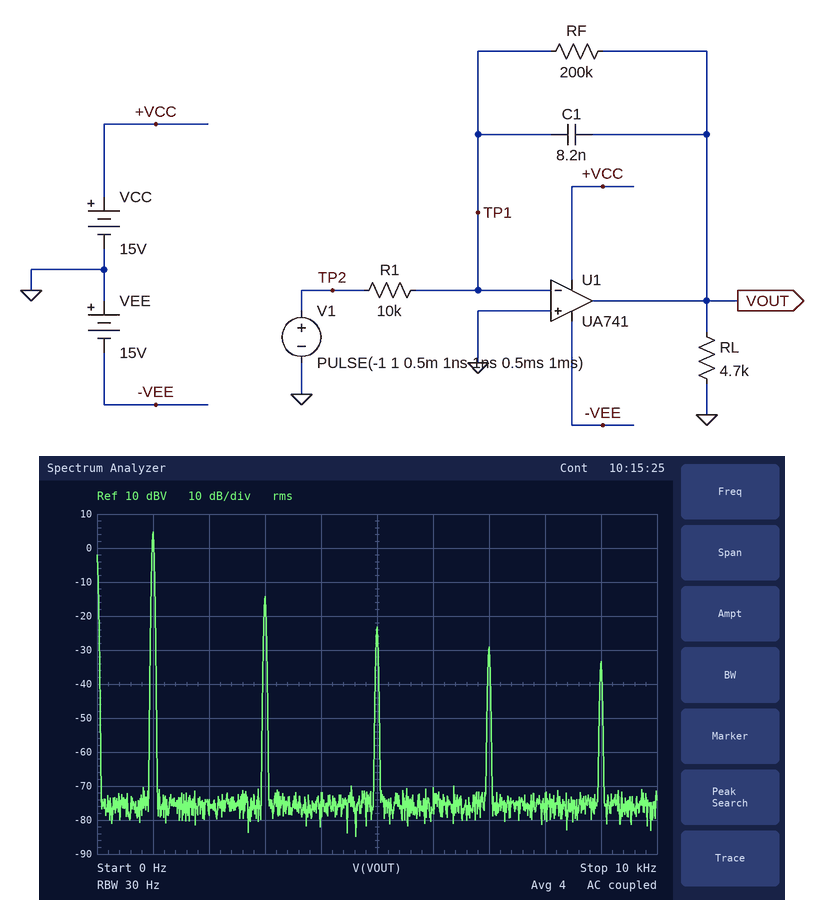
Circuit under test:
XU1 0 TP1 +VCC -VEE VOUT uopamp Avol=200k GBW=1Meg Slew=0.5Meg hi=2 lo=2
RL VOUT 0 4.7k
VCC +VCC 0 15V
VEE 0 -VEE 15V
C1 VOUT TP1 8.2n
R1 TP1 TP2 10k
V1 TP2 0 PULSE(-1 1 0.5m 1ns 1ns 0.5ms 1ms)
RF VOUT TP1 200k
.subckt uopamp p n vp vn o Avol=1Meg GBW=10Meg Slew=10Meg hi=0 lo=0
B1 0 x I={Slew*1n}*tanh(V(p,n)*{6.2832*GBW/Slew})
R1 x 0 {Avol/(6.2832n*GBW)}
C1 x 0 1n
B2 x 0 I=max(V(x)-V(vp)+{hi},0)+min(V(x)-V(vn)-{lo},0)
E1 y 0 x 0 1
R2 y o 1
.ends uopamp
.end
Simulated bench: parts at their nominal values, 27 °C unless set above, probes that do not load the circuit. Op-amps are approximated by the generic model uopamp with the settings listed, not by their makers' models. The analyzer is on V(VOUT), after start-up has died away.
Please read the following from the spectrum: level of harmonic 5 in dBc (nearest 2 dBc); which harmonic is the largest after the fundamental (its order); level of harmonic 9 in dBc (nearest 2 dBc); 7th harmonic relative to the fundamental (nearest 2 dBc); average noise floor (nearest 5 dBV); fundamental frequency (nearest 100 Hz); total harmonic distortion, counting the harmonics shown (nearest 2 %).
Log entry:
-28 dBc
3
-38 dBc
-34 dBc
-75 dBV
1.0 kHz
12 %
